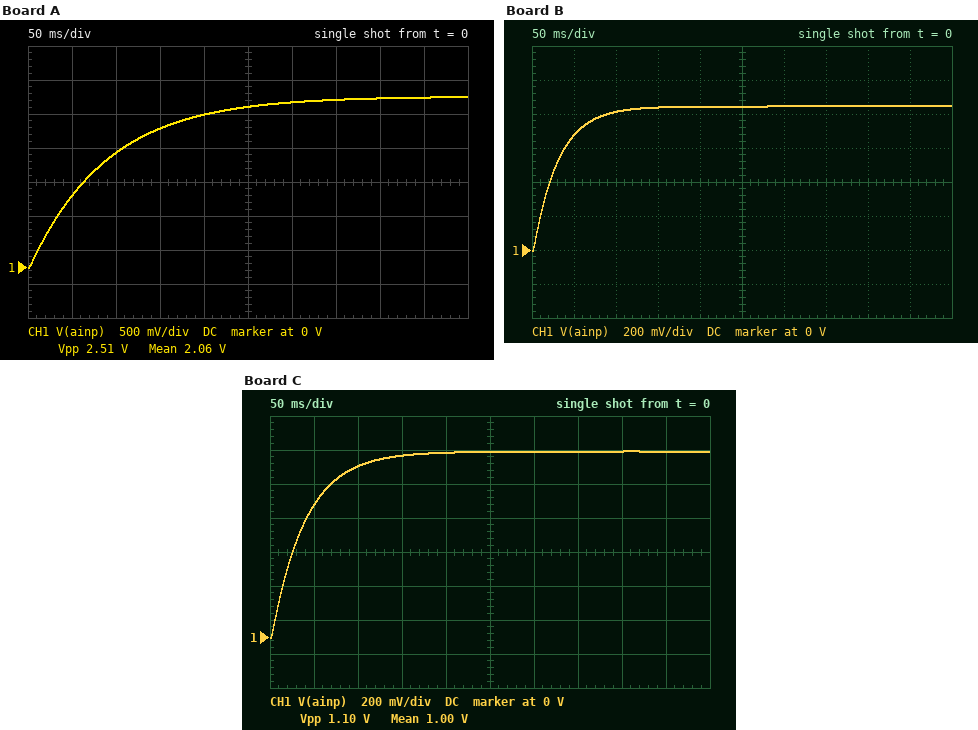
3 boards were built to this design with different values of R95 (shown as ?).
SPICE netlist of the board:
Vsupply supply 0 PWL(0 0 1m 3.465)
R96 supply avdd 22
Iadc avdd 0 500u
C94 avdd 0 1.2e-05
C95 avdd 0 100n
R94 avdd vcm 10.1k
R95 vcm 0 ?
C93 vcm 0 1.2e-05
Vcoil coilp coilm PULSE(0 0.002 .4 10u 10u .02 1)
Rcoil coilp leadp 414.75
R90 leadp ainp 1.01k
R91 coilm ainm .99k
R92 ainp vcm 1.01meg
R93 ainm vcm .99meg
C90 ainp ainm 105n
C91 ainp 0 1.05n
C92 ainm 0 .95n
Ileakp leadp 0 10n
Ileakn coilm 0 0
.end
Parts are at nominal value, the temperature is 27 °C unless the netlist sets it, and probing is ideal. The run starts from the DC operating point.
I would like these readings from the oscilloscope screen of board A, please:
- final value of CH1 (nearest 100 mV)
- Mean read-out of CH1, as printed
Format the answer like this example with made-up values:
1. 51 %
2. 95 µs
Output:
1. 2.5 V
2. 2.06 V
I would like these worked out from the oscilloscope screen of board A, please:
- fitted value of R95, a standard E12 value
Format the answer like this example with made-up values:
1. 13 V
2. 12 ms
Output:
1. 27 kΩ
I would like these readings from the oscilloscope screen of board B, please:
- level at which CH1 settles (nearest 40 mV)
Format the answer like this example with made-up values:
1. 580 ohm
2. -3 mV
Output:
1. 840 mV
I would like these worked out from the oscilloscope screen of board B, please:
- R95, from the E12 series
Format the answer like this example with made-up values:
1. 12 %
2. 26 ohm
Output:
1. 3.3 kΩ
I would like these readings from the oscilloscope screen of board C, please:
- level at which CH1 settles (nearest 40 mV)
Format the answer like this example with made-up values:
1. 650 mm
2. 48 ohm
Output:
1. 1.08 V
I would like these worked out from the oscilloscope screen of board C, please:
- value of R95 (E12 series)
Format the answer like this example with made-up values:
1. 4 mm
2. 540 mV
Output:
1. 4.7 kΩ
